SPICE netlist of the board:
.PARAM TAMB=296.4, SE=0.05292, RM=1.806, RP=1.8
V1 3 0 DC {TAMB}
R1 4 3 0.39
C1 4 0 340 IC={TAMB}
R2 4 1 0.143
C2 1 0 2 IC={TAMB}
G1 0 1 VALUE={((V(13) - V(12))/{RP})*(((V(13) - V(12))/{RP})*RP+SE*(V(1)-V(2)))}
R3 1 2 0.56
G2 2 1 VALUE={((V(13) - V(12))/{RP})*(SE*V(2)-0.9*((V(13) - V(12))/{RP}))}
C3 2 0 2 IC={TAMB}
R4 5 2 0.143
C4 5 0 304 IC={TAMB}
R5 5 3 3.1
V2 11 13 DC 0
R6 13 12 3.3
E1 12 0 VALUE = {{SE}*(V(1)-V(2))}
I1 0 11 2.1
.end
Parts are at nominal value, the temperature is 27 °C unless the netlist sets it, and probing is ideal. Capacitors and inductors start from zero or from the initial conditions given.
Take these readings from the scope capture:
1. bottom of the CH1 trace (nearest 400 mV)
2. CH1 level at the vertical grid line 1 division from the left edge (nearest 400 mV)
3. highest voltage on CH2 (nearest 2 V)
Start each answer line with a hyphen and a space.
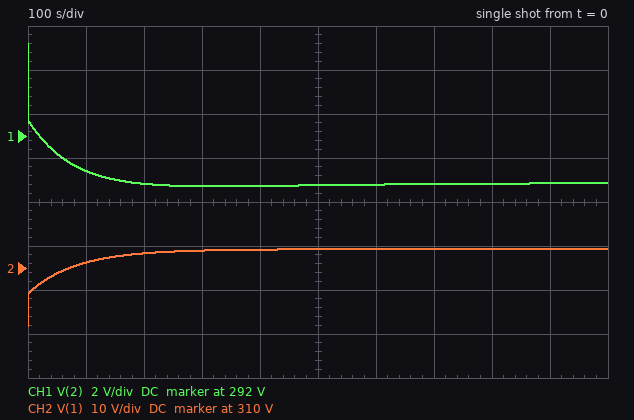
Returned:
- 289.6 V
- 290.4 V
- 314 V
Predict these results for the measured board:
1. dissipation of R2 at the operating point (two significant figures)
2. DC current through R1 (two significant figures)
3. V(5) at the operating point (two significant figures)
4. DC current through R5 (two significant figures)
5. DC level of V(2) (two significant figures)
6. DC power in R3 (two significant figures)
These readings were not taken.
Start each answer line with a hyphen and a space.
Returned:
- 160 W
- 34 A
- 290 V
- 2.0 A
- 290 V
- 1.1 kW
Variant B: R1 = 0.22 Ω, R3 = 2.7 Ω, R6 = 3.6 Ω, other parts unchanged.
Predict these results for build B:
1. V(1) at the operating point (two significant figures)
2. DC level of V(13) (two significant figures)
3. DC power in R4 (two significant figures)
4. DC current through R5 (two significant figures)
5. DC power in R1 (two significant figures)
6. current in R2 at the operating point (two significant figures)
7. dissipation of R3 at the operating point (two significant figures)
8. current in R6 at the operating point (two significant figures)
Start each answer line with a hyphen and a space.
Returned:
- 320 V
- 11 V
- 29 W
- 14 A
- 830 W
- 61 A
- 1.7 kW
- 2.1 A
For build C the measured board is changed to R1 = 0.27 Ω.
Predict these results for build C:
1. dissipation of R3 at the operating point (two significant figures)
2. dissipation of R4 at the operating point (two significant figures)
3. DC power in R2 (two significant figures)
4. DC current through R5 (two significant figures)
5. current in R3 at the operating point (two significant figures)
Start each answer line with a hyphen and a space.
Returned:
- 1.0 kW
- 1.2 W
- 170 W
- 2.9 A
- 42 A
